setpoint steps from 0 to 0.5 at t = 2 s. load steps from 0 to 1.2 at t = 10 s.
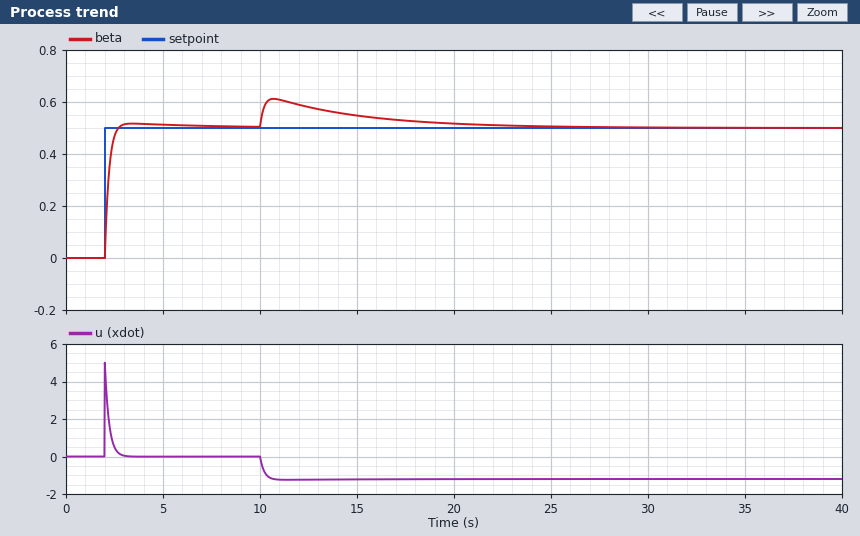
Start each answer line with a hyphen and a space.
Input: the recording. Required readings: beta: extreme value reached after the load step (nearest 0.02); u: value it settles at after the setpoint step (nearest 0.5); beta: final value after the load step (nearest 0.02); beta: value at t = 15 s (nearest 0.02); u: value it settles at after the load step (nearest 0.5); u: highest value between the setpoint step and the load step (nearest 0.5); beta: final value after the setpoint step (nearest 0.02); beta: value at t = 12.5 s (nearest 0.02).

- 0.62
- 0.0
- 0.50
- 0.54
- -1.0
- 5.0
- 0.50
- 0.58
